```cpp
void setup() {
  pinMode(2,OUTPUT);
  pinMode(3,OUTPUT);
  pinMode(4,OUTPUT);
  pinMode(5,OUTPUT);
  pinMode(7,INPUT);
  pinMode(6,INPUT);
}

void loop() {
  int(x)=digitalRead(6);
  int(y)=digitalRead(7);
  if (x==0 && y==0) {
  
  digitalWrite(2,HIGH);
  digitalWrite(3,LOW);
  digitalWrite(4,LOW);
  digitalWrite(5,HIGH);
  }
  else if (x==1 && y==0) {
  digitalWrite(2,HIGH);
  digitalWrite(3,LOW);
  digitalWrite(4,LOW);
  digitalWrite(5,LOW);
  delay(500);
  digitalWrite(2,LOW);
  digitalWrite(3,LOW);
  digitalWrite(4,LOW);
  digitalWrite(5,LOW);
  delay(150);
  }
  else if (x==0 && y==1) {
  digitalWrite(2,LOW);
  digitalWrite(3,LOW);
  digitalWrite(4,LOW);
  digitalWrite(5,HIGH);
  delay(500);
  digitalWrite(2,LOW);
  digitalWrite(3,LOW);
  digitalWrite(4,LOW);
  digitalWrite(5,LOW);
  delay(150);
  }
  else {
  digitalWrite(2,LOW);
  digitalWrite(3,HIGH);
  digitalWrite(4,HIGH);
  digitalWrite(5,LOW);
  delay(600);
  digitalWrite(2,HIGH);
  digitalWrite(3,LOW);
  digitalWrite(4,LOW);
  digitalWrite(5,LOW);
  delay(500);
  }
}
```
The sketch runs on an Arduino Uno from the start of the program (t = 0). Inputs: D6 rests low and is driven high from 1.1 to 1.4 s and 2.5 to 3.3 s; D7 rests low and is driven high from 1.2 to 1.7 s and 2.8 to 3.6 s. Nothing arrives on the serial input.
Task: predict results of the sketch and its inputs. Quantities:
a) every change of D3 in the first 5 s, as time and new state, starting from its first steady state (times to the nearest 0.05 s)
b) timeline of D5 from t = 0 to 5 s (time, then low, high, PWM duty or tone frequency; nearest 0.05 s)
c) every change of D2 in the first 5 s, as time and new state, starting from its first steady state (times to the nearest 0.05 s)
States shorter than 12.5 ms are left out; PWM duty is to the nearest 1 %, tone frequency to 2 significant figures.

0 s low; 3.15 s high; 3.75 s low
0 s high; 1.1 s low; 1.75 s high; 2.5 s low; 4.25 s high
0 s high; 1.6 s low; 1.75 s high; 3 s low; 3.75 s high
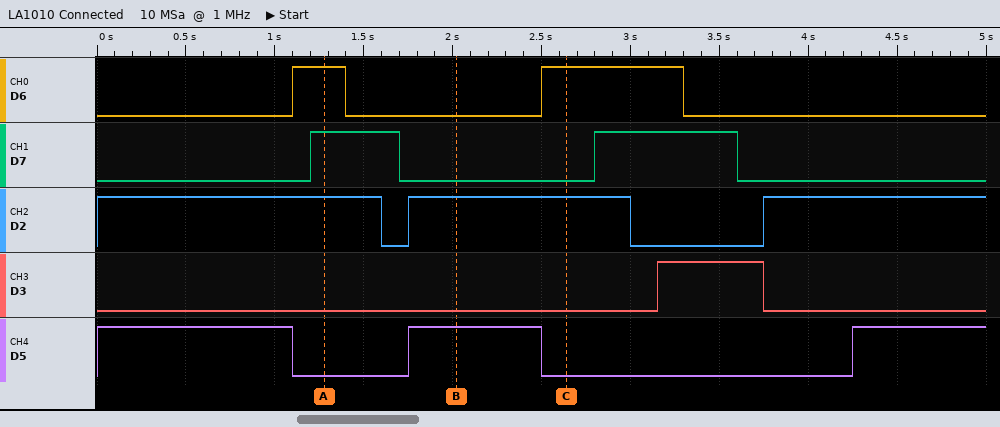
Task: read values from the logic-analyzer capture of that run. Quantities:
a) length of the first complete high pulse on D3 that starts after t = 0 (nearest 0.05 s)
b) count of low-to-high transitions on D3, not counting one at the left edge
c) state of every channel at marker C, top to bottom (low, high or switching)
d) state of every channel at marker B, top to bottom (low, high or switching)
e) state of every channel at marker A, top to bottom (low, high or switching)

0.60 s
1
D6 high, D7 low, D2 high, D3 low, D5 low
D6 low, D7 low, D2 high, D3 low, D5 high
D6 high, D7 high, D2 high, D3 low, D5 low
